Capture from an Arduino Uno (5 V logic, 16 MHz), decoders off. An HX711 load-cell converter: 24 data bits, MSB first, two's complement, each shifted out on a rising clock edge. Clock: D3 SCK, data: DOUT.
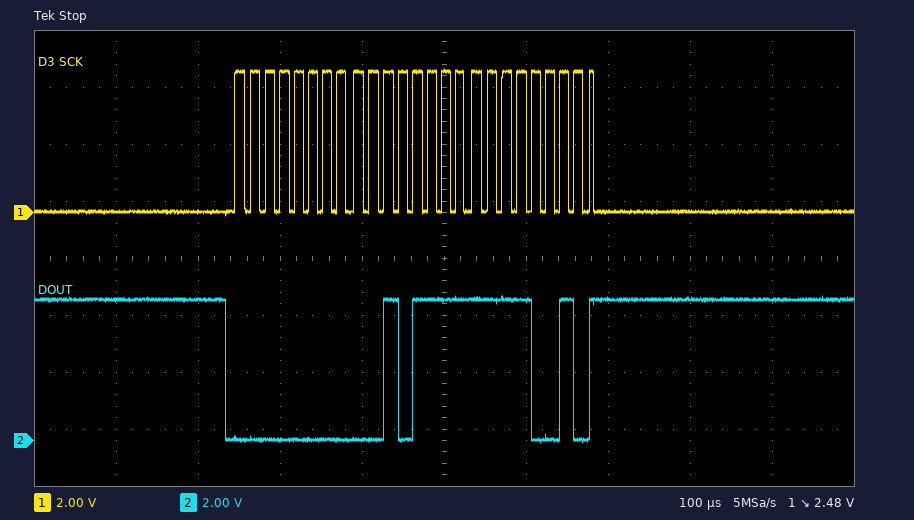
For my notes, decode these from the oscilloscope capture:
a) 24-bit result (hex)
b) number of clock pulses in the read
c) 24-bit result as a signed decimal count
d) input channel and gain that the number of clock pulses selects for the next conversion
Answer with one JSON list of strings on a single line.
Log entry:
["0x002FF2", "25", "12274", "channel A, gain 128"]
